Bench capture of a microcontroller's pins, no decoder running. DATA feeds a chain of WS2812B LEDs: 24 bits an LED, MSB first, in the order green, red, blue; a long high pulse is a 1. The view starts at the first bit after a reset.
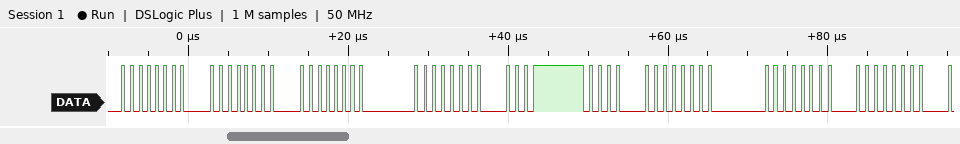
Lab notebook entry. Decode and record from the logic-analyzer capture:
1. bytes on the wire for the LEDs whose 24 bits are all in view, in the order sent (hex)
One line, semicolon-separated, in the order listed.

00 00 00 00 10 00
